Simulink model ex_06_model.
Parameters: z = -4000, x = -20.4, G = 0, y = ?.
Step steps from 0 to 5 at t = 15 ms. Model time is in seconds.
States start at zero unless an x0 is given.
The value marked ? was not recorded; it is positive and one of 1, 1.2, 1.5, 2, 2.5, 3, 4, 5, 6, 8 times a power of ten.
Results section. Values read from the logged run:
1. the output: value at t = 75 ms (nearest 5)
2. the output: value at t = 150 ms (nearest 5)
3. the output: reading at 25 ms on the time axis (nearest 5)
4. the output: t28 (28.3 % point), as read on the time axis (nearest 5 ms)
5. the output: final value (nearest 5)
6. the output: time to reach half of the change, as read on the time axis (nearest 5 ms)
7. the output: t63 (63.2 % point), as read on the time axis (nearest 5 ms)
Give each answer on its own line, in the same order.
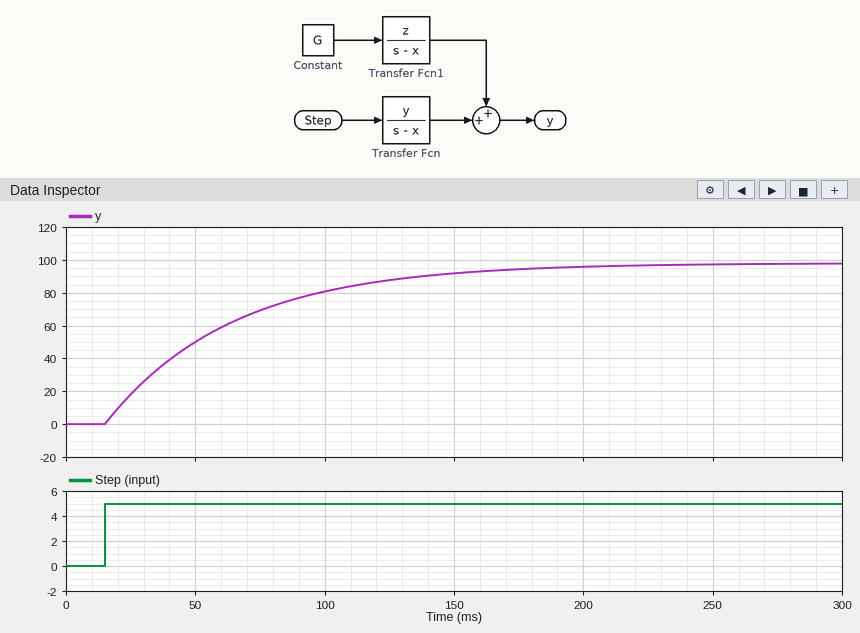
70
90
20
30 ms
100
50 ms
65 ms
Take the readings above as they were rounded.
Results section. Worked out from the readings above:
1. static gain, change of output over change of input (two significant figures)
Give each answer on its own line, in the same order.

20
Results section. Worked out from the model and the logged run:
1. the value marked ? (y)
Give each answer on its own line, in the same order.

400
